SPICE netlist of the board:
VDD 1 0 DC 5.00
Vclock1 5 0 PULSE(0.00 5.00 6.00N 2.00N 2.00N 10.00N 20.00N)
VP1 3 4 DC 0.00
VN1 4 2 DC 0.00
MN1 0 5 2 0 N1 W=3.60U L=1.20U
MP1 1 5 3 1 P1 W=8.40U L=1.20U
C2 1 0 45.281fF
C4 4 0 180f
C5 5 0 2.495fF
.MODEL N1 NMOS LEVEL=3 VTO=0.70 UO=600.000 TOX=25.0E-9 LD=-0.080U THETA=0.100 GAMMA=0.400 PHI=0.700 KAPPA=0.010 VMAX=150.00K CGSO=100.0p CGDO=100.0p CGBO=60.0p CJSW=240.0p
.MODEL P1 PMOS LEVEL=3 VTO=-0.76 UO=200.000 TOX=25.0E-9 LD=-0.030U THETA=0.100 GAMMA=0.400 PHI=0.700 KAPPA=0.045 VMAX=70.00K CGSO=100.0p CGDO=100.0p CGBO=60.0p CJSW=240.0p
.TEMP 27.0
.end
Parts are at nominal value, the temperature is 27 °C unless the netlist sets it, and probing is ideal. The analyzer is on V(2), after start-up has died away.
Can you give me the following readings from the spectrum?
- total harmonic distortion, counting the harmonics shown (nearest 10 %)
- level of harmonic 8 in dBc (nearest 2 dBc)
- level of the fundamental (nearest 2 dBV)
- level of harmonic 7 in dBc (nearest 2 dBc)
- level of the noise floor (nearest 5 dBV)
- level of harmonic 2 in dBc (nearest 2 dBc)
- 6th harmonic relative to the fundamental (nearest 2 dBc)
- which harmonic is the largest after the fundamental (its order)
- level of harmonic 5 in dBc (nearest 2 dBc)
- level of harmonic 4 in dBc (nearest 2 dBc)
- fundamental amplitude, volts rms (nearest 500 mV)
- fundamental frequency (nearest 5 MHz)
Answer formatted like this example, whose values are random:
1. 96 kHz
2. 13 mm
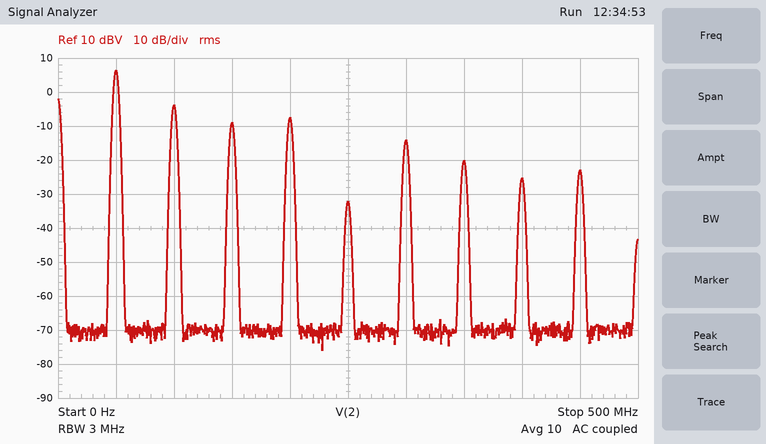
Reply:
1. 40 %
2. -32 dBc
3. 6 dBV
4. -26 dBc
5. -70 dBV
6. -10 dBc
7. -20 dBc
8. 2
9. -38 dBc
10. -14 dBc
11. 2.0 V
12. 50 MHz
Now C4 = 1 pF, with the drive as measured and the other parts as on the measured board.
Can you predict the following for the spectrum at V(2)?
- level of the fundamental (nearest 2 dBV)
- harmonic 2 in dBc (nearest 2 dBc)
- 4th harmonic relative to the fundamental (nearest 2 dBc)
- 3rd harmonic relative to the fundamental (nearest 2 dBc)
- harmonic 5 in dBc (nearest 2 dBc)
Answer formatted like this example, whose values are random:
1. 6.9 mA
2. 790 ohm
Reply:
1. 4 dBV
2. -14 dBc
3. -28 dBc
4. -28 dBc
5. -46 dBc
